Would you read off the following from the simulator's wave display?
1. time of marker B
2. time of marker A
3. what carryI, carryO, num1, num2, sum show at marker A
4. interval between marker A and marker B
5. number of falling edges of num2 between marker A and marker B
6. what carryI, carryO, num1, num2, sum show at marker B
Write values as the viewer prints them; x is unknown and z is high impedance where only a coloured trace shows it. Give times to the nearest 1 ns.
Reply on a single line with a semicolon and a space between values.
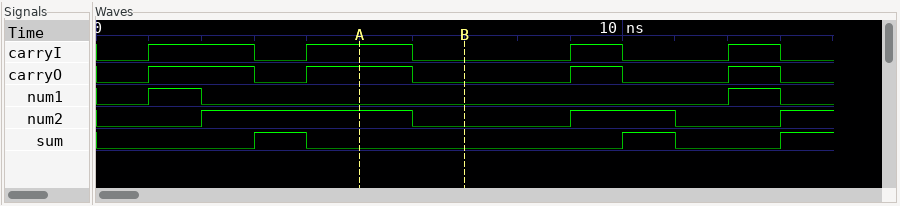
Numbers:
7 ns; 5 ns; carryI=1, carryO=1, num1=0, num2=1, sum=0; 2 ns; 1; carryI=0, carryO=0, num1=0, num2=0, sum=0
